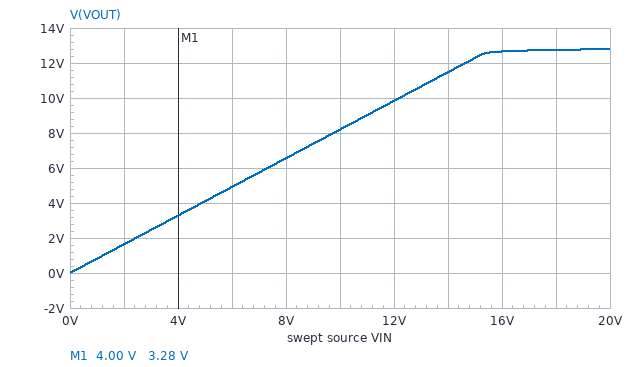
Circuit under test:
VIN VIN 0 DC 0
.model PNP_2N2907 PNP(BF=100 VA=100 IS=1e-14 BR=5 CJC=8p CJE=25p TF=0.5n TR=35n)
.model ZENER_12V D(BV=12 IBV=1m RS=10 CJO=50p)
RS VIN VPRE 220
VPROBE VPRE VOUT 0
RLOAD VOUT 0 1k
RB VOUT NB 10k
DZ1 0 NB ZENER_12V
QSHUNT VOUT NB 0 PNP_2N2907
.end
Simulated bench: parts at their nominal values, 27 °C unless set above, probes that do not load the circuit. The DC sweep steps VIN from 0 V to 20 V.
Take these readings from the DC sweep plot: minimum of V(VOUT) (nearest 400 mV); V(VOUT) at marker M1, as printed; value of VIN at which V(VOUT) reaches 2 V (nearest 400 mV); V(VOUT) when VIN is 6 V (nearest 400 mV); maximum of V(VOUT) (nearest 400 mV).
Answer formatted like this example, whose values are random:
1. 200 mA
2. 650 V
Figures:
1. 0 V
2. 3.28 V
3. 2.4 V
4. 4.8 V
5. 12.8 V
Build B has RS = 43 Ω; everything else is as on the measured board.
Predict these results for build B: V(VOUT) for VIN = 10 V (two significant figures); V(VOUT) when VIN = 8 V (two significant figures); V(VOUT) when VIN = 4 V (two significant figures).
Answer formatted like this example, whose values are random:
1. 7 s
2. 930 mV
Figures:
1. 9.6 V
2. 7.7 V
3. 3.8 V
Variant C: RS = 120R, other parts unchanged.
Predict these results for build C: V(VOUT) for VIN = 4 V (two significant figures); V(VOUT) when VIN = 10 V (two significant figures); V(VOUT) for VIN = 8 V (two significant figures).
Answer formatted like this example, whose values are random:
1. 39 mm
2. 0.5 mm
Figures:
1. 3.6 V
2. 8.9 V
3. 7.1 V
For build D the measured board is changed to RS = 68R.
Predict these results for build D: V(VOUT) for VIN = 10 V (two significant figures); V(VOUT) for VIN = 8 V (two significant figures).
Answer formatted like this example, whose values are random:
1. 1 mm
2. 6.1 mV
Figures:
1. 9.4 V
2. 7.5 V
